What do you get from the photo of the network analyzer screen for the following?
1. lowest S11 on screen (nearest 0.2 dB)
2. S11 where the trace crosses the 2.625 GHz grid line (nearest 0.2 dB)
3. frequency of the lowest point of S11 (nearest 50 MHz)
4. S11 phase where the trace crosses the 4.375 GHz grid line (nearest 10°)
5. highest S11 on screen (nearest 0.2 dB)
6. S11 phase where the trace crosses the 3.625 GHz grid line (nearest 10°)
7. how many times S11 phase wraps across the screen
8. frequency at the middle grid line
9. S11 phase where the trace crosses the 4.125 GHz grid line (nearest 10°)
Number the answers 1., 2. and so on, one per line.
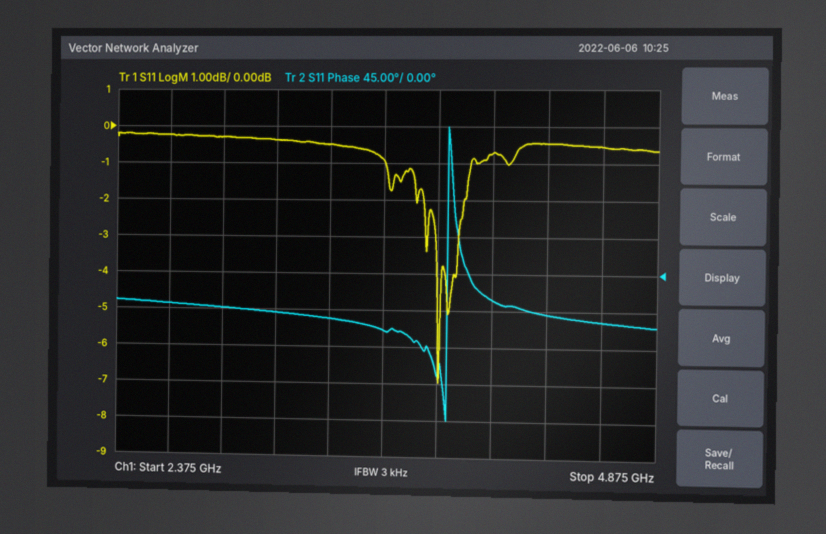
1. -7.0 dB
2. -0.2 dB
3. 3.90 GHz
4. -50°
5. -0.2 dB
6. -70°
7. 1
8. 3.625 GHz
9. -30°
